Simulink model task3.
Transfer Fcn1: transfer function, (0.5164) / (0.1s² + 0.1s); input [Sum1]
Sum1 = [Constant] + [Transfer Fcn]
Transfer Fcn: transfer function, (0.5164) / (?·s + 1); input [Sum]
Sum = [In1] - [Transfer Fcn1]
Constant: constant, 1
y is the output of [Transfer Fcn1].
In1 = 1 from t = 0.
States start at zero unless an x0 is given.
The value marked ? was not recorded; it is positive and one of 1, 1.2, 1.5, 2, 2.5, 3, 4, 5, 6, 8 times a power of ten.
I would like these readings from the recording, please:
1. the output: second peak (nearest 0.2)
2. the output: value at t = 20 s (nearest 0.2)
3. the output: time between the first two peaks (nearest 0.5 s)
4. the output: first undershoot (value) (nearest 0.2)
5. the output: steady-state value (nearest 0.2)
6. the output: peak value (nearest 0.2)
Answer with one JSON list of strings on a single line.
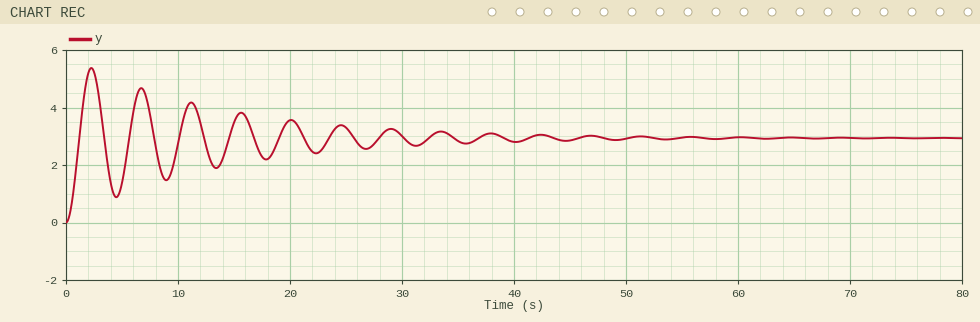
["4.6", "3.6", "4.5 s", "0.8", "3.0", "5.4"]
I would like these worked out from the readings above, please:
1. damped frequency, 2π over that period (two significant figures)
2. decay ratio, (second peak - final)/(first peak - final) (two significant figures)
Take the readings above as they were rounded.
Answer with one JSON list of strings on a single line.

["1.4 rad/s", "0.67"]
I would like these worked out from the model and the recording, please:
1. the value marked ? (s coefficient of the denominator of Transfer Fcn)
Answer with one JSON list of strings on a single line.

["0.4"]
